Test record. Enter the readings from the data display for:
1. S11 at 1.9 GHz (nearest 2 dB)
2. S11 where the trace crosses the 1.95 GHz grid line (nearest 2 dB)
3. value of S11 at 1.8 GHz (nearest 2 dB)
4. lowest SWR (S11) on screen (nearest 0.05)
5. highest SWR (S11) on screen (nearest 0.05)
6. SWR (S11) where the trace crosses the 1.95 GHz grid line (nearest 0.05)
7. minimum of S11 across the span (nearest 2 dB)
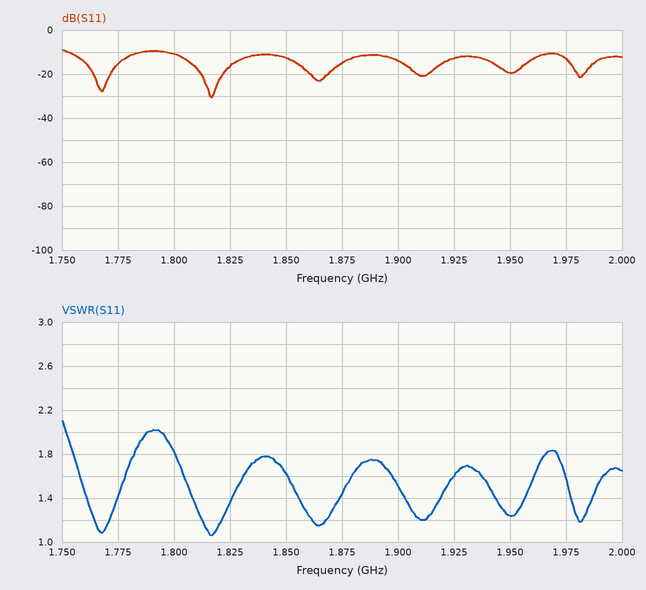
-14 dB
-20 dB
-10 dB
1.05
2.10
1.25
-30 dB
